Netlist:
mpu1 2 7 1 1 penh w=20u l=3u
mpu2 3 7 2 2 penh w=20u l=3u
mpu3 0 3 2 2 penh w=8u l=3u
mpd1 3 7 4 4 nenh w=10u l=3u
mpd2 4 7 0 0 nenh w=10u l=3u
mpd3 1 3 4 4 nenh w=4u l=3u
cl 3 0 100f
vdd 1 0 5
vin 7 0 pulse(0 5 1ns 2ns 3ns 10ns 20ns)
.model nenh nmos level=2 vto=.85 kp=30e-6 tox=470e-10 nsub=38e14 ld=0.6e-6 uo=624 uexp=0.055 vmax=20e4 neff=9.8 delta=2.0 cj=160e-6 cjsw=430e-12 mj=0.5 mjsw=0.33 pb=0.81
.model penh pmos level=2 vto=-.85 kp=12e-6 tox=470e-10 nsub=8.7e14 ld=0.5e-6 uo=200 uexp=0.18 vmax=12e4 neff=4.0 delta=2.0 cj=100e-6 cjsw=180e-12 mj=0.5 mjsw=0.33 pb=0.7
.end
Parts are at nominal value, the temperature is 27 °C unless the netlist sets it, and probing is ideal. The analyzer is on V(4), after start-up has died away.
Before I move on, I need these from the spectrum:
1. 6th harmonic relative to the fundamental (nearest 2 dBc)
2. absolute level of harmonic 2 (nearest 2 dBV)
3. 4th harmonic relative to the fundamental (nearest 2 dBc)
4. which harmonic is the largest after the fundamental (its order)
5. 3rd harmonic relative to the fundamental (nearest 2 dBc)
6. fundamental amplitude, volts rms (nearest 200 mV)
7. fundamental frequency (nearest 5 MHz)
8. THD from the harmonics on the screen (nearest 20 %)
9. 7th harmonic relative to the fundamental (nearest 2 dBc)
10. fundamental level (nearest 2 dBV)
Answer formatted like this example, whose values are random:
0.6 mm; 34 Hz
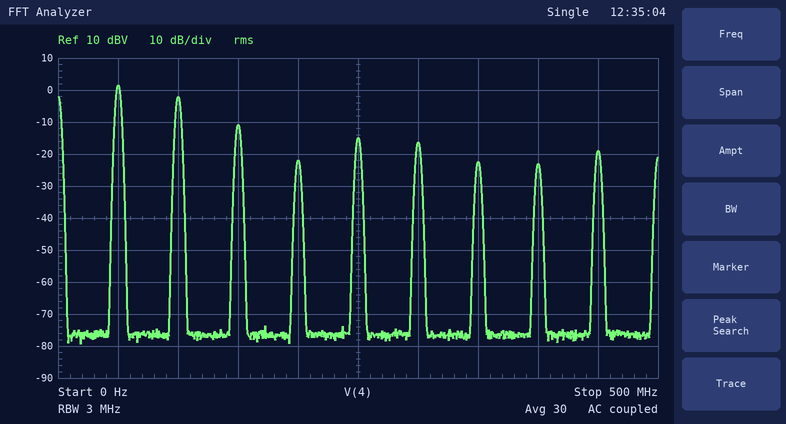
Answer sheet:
-18 dBc; -2 dBV; -24 dBc; 2; -12 dBc; 1.2 V; 50 MHz; 80 %; -24 dBc; 2 dBV
